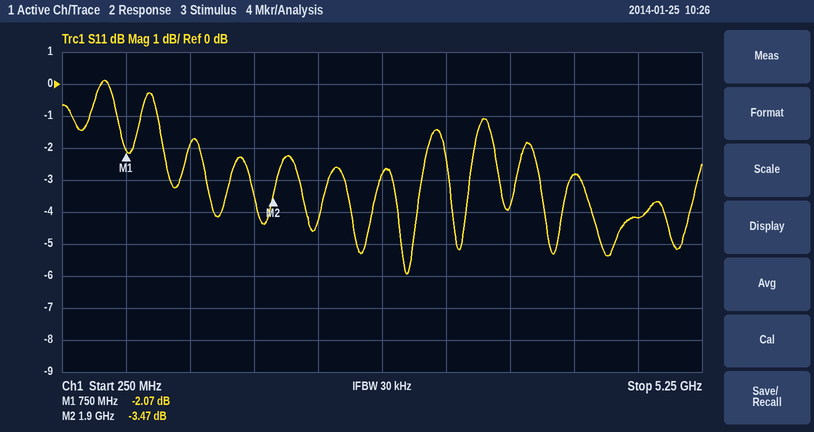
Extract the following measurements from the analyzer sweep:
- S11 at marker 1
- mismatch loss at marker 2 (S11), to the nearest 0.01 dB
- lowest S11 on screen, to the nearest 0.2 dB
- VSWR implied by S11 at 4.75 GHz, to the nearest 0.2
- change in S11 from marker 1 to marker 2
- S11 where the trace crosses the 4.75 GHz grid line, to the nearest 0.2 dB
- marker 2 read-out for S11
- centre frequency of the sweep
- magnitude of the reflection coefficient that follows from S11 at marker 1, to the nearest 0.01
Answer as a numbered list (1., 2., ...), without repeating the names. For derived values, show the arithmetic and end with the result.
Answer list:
1. -2.07 dB
2. −10 log10(1 − 10^(-3.47/10)) ≈ 2.59 dB
3. -6.0 dB
4. |Γ| = 10^(-4.2/20) = 0.6166; VSWR = (1 + 0.6166)/(1 − 0.6166) ≈ 4.2
5. -3.47 − (-2.07) = -1.40 dB
6. -4.2 dB
7. -3.47 dB
8. 2.75 GHz
9. 10^(-2.07/20) ≈ 0.79
